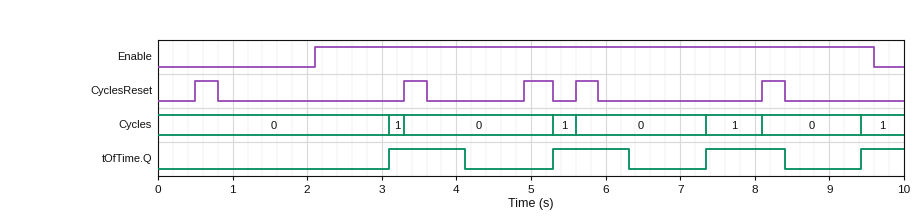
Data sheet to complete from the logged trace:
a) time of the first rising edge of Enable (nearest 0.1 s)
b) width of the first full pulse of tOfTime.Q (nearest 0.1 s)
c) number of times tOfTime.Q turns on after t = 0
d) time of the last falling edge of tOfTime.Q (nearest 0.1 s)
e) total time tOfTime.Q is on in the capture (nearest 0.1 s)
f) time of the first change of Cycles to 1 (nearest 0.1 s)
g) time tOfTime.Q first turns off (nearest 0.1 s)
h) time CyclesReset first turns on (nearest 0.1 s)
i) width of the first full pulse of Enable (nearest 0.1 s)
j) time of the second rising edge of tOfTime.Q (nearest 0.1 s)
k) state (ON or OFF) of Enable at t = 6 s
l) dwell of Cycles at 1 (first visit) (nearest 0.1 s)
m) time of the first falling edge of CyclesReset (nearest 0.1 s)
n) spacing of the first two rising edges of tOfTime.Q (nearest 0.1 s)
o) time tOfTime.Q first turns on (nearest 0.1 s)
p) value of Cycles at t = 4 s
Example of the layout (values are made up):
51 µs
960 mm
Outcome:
2.1 s
1.0 s
4
8.4 s
3.7 s
3.1 s
4.1 s
0.5 s
7.5 s
5.3 s
ON
0.2 s
0.8 s
2.2 s
3.1 s
0
